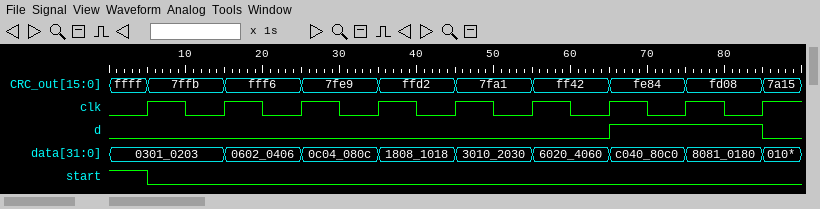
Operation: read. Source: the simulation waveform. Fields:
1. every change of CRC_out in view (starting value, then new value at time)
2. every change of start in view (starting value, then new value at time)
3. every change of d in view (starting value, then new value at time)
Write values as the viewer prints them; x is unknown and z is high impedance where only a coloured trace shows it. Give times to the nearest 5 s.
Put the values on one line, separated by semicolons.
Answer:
ffff, 7ffb at 5 s, fff6 at 15 s, 7fe9 at 25 s, ffd2 at 35 s, 7fa1 at 45 s, ff42 at 55 s, fe84 at 65 s, fd08 at 75 s, 7a15 at 85 s; 1, 0 at 5 s; 0, 1 at 65 s, 0 at 85 s
